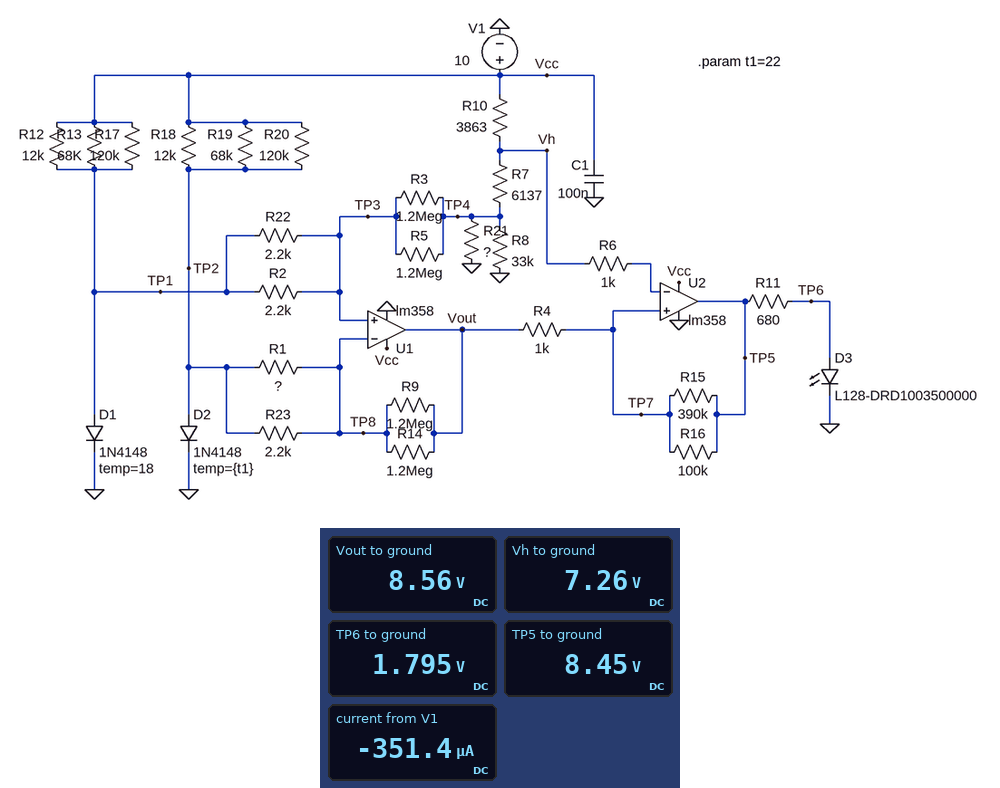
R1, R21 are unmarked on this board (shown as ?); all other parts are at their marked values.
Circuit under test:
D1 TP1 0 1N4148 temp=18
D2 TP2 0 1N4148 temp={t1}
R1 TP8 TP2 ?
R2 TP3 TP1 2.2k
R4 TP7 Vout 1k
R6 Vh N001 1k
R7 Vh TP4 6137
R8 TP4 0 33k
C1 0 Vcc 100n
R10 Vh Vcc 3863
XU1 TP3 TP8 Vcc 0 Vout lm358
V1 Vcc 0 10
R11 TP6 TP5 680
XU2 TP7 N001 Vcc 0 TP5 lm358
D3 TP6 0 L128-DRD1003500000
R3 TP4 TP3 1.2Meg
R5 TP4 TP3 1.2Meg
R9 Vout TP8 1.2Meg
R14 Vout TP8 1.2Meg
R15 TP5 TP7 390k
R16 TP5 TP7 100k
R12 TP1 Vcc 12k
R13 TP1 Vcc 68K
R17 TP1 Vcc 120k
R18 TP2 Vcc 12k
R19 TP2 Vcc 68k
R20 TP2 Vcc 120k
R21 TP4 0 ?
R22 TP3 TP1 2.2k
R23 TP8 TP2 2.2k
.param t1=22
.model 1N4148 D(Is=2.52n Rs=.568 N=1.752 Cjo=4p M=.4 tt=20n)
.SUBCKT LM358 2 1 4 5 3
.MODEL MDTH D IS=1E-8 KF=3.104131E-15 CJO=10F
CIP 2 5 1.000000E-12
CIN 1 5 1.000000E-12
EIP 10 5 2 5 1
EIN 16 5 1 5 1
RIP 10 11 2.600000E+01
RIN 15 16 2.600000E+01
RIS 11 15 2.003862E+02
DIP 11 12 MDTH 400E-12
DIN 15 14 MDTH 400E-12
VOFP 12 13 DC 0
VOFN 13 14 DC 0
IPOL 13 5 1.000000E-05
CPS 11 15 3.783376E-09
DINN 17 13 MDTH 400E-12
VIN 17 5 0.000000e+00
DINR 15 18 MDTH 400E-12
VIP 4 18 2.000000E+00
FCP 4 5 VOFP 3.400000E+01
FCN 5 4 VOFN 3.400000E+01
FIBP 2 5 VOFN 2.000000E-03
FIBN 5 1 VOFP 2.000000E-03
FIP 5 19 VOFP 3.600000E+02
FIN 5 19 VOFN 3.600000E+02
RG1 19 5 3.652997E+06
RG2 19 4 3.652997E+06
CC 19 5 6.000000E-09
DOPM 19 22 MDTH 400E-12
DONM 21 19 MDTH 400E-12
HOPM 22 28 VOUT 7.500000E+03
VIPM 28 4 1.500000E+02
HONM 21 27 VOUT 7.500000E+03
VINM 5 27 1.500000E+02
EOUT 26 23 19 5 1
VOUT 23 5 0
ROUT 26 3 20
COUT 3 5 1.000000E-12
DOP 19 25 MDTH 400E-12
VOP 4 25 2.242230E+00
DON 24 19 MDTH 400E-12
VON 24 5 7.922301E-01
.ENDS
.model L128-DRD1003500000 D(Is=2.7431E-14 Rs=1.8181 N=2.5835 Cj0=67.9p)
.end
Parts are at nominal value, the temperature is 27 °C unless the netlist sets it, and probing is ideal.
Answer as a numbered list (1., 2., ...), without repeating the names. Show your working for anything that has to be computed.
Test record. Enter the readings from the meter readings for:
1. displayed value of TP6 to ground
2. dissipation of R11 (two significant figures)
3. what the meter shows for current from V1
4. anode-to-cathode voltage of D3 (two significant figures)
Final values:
1. 1.795 V
2. (8.45 V - 1.795 V)^2 / 680 Ω = 65 mW
3. -351.4 µA
4. 1.795 V = 1.8 V
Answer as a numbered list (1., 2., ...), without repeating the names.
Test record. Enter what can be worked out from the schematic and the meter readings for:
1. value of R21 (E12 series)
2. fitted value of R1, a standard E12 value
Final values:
1. 4.7 kΩ
2. 1 kΩ
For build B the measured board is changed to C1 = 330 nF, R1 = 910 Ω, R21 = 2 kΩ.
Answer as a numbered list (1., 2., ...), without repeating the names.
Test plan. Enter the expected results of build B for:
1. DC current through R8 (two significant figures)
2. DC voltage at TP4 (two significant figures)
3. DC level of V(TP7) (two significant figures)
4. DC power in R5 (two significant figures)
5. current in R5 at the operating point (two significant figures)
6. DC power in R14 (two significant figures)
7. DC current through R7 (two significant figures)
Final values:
1. 48 µA
2. 1.6 V
3. 8.5 V
4. 800 nW
5. 820 nA
6. 52 µW
7. 840 µA
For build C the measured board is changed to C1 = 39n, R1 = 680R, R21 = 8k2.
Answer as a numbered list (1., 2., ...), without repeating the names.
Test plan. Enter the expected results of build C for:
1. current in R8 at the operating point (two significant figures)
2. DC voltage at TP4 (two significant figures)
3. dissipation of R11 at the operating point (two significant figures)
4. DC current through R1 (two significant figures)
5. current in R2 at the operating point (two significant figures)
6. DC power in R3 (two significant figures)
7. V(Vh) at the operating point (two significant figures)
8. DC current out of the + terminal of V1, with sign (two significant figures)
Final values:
1. 120 µA
2. 3.9 V
3. 65 mW
4. 10 µA
5. 2.8 µA
6. 9.3 µW
7. 7.7 V
8. -680 µA
